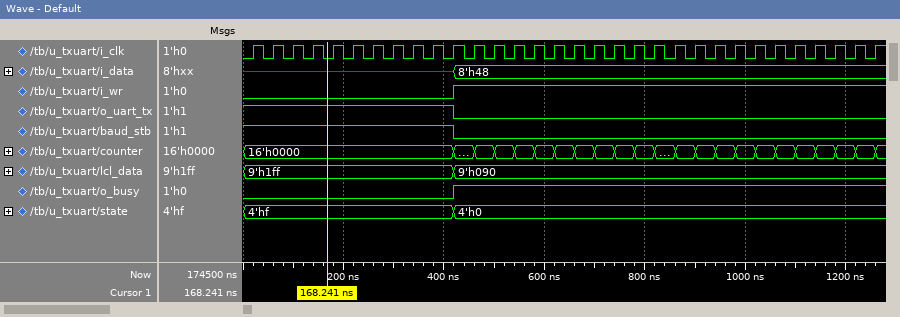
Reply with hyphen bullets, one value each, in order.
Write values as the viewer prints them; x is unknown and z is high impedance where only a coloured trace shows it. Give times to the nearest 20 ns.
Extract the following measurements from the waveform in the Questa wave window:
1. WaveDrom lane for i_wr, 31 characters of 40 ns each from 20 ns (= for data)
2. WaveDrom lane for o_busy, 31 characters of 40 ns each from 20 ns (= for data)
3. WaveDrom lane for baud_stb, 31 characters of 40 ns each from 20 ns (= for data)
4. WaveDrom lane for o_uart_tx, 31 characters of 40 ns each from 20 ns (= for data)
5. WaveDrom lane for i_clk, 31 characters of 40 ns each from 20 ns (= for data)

- {name: 'i_wr', wave: '0.........1....................'}
- {name: 'o_busy', wave: '0.........1....................'}
- {name: 'baud_stb', wave: '1.........0....................'}
- {name: 'o_uart_tx', wave: '1.........0....................'}
- {name: 'i_clk', wave: 'p..............................'}
